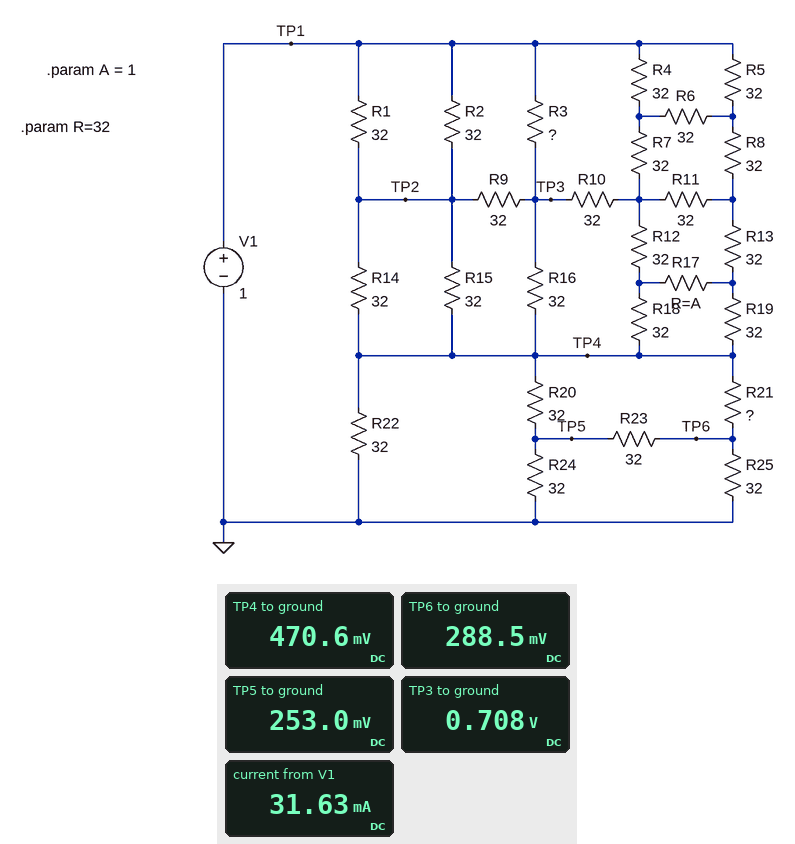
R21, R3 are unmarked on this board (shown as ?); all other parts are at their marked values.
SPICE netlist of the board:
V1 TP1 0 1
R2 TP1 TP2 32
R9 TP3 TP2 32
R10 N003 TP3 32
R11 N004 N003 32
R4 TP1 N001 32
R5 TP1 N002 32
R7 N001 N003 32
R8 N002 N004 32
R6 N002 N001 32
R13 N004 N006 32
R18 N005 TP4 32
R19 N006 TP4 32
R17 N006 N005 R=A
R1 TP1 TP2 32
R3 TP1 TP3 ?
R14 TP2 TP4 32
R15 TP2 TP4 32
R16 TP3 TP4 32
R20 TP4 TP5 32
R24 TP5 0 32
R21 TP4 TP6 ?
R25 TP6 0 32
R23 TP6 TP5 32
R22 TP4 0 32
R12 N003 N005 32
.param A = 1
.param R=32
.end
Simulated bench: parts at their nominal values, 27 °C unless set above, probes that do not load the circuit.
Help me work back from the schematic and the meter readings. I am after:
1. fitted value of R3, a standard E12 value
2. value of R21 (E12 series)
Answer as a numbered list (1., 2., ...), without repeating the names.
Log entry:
1. 47 Ω
2. 18 Ω
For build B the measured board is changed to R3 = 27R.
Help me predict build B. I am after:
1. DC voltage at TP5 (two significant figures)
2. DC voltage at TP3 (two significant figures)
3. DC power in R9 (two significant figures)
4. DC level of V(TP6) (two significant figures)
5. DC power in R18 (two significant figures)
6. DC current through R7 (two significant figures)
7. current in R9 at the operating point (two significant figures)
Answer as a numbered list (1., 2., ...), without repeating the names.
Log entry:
1. 260 mV
2. 760 mV
3. 3.5 µW
4. 300 mV
5. 530 µW
6. 3.9 mA
7. 330 µA
